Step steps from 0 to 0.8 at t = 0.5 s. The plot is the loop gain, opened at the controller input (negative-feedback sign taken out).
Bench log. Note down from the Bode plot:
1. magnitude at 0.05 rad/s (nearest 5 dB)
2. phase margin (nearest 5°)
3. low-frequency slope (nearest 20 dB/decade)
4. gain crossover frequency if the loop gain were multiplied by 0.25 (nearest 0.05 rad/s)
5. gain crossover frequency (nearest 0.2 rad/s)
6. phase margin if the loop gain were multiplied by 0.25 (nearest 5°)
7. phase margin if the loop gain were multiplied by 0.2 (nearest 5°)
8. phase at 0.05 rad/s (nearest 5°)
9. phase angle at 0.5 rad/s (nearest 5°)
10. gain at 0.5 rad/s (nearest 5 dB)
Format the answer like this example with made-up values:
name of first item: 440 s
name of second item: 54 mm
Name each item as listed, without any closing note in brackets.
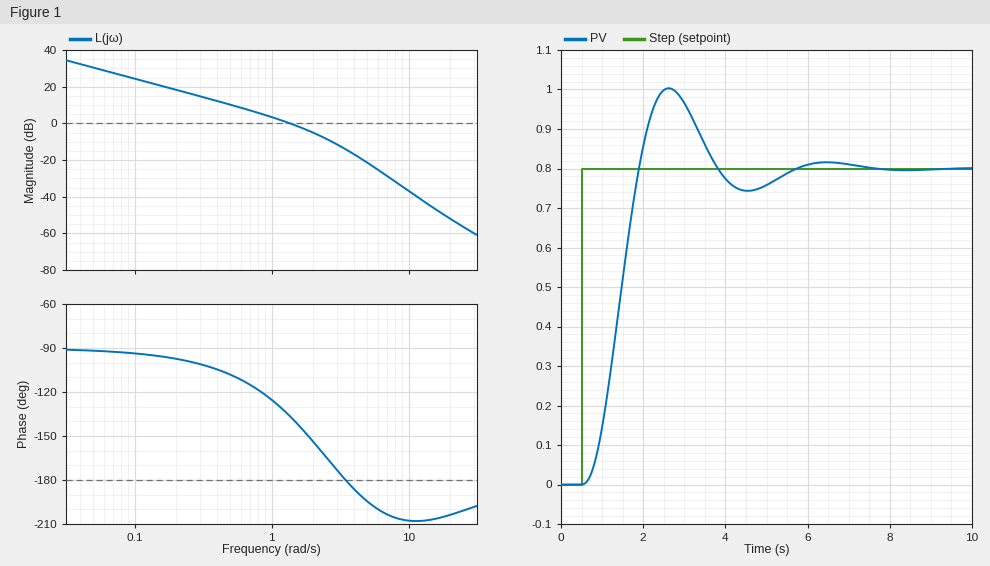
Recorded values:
magnitude at 0.05 rad/s: 30 dB
phase margin: 45°
low-frequency slope: -20 dB/decade
gain crossover frequency if the loop gain were multiplied by 0.25: 0.40 rad/s
gain crossover frequency: 1.4 rad/s
phase margin if the loop gain were multiplied by 0.25: 75°
phase margin if the loop gain were multiplied by 0.2: 80°
phase at 0.05 rad/s: -90°
phase angle at 0.5 rad/s: -110°
gain at 0.5 rad/s: 10 dB
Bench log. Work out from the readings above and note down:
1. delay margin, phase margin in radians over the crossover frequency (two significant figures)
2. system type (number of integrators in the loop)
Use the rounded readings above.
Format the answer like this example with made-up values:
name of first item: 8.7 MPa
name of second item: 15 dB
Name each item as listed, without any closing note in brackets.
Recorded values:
delay margin, phase margin in radians over the crossover frequency: 0.56 s
system type: 1
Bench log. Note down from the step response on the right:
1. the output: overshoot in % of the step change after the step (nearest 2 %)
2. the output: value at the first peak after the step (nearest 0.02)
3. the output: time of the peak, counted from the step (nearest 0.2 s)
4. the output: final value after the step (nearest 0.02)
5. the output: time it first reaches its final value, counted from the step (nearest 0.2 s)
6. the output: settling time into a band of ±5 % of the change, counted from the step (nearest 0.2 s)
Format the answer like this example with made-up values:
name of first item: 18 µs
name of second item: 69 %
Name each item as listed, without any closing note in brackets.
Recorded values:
the output: overshoot in % of the step change after the step: 26 %
the output: value at the first peak after the step: 1.00
the output: time of the peak, counted from the step: 2.2 s
the output: final value after the step: 0.80
the output: time it first reaches its final value, counted from the step: 1.4 s
the output: settling time into a band of ±5 % of the change, counted from the step: 4.6 s
